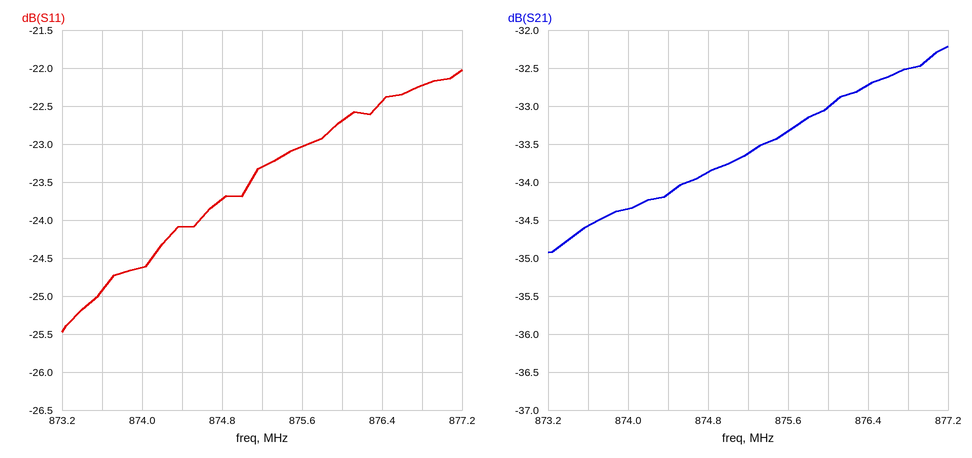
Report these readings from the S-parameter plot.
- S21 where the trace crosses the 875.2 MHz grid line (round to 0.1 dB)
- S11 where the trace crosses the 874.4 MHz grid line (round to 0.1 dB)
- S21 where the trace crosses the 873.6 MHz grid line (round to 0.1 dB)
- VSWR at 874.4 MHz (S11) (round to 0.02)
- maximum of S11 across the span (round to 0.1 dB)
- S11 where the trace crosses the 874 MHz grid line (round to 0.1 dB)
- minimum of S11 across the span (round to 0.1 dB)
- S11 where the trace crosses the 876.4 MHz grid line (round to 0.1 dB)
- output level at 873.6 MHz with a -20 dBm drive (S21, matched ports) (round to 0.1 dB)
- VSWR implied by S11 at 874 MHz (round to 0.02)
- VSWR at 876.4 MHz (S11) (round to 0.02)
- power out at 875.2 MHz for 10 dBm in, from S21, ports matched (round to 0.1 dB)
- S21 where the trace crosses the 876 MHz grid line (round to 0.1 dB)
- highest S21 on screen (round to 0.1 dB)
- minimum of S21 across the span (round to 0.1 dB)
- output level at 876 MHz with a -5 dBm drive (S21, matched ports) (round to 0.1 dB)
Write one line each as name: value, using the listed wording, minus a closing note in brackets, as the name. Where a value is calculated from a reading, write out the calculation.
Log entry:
S21 where the trace crosses the 875.2 MHz grid line: -33.6 dB
S11 where the trace crosses the 874.4 MHz grid line: -24.1 dB
S21 where the trace crosses the 873.6 MHz grid line: -34.6 dB
VSWR at 874.4 MHz (S11): |Γ| = 10^(-24.1/20) = 0.0624; VSWR = (1 + 0.0624)/(1 − 0.0624) ≈ 1.13, so 1.14 to the nearest 0.02
maximum of S11 across the span: -22.0 dB
S11 where the trace crosses the 874 MHz grid line: -24.6 dB
minimum of S11 across the span: -25.5 dB
S11 where the trace crosses the 876.4 MHz grid line: -22.4 dB
output level at 873.6 MHz with a -20 dBm drive (S21, matched ports): -20 dBm + (-34.6 dB) = -54.6 dBm
VSWR implied by S11 at 874 MHz: |Γ| = 10^(-24.6/20) = 0.0589; VSWR = (1 + 0.0589)/(1 − 0.0589) ≈ 1.13, so 1.12 to the nearest 0.02
VSWR at 876.4 MHz (S11): |Γ| = 10^(-22.4/20) = 0.0759; VSWR = (1 + 0.0759)/(1 − 0.0759) ≈ 1.16
power out at 875.2 MHz for 10 dBm in, from S21, ports matched: 10 dBm + (-33.6 dB) = -23.6 dBm
S21 where the trace crosses the 876 MHz grid line: -33.0 dB
highest S21 on screen: -32.2 dB
minimum of S21 across the span: -34.9 dB
output level at 876 MHz with a -5 dBm drive (S21, matched ports): -5 dBm + (-33.0 dB) = -38.0 dBm
